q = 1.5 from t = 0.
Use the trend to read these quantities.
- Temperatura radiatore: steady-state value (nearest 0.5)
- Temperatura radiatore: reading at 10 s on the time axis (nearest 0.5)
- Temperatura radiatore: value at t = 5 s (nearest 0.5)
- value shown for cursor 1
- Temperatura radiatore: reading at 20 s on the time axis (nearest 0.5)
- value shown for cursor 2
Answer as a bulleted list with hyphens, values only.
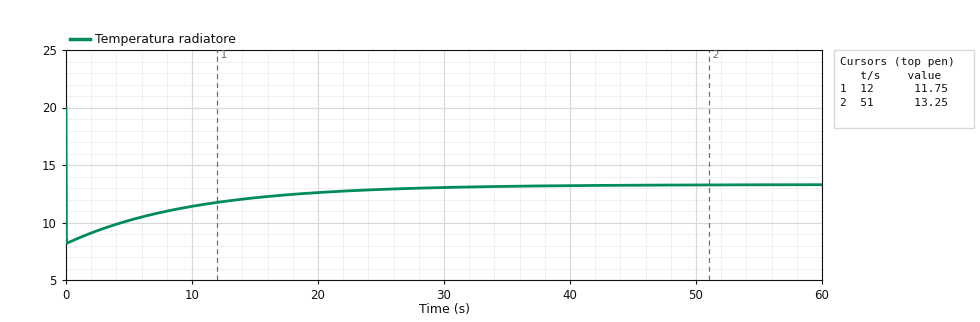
- 13.5
- 11.5
- 10.0
- 11.75
- 12.5
- 13.25
